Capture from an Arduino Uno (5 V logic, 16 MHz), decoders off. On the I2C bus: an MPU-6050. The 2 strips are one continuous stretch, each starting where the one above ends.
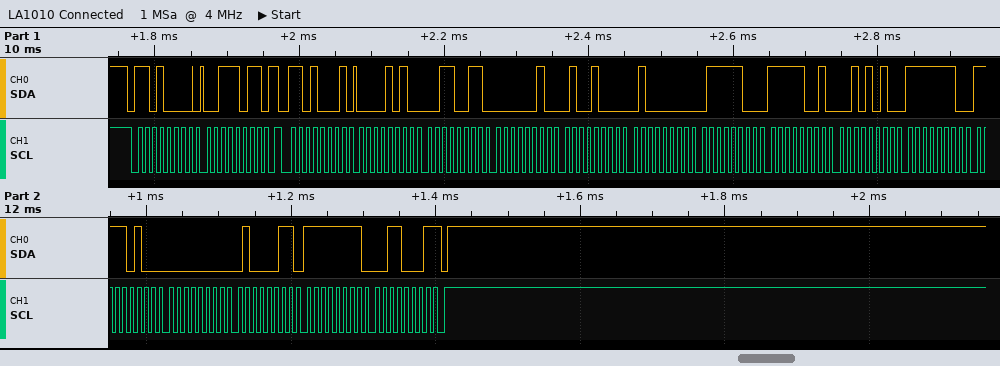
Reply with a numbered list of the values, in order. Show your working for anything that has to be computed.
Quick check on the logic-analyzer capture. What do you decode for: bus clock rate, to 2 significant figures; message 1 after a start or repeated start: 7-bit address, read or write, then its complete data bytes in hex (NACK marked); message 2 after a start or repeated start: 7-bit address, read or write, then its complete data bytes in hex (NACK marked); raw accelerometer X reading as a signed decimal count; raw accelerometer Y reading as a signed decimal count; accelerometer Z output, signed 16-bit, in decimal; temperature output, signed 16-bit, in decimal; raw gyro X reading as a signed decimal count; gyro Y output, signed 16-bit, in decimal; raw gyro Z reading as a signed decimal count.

1. 100 kHz
2. 0x68 write: 3B
3. 0x68 read: 0A 33 02 48 40 7C F9 2A FE F4 00 43 FF 31 NACK
4. 0x0A33 = 2611
5. 0x0248 = 584
6. 0x407C = 16508
7. 0xF92A = -1750
8. 0xFEF4 = -268
9. 0x0043 = 67
10. 0xFF31 = -207
